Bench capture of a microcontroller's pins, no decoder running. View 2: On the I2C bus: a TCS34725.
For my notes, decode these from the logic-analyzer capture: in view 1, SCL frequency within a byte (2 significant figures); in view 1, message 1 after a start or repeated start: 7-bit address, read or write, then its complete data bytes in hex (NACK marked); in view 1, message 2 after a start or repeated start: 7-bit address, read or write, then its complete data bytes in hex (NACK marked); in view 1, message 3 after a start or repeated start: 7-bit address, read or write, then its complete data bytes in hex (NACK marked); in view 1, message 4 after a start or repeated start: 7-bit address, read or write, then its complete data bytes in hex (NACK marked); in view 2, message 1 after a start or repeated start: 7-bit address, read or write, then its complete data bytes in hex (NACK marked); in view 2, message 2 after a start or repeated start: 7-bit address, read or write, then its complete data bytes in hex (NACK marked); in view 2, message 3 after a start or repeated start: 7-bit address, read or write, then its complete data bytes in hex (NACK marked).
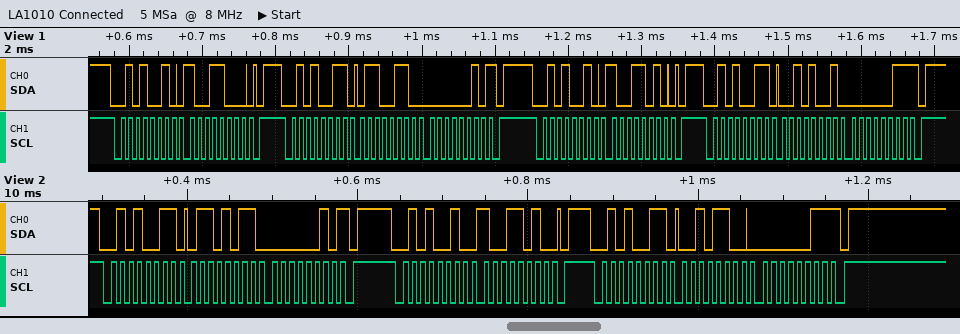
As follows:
100 kHz
0x29 write: 98
0x29 read: 66 02 NACK
0x29 write: 9A
0x29 read: 29 03 NACK
0x29 read: 6B 02 NACK
0x29 write: 9A
0x29 read: 2C 03 NACK
